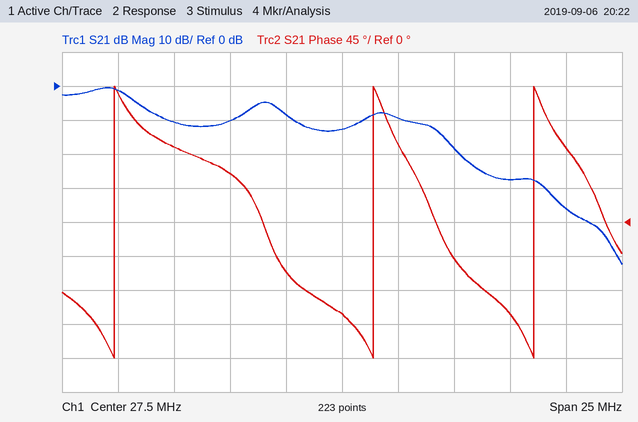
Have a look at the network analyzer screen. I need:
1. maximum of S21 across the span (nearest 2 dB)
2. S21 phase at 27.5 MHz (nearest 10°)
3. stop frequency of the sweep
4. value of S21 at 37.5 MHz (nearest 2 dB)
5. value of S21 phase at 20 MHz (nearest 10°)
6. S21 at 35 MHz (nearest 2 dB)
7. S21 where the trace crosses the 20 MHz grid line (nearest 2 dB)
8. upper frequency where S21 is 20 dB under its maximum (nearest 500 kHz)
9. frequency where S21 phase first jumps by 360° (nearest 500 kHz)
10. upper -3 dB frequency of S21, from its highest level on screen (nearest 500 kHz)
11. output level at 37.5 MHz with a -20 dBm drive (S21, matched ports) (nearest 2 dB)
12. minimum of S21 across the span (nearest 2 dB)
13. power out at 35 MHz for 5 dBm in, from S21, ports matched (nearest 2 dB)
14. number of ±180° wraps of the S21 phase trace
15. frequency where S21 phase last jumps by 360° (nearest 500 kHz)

0 dB
-120°
40 MHz
-36 dB
100°
-28 dB
-10 dB
33.0 MHz
17.5 MHz
18.0 MHz
-56 dBm
-52 dB
-22 dBm
3
36.0 MHz
